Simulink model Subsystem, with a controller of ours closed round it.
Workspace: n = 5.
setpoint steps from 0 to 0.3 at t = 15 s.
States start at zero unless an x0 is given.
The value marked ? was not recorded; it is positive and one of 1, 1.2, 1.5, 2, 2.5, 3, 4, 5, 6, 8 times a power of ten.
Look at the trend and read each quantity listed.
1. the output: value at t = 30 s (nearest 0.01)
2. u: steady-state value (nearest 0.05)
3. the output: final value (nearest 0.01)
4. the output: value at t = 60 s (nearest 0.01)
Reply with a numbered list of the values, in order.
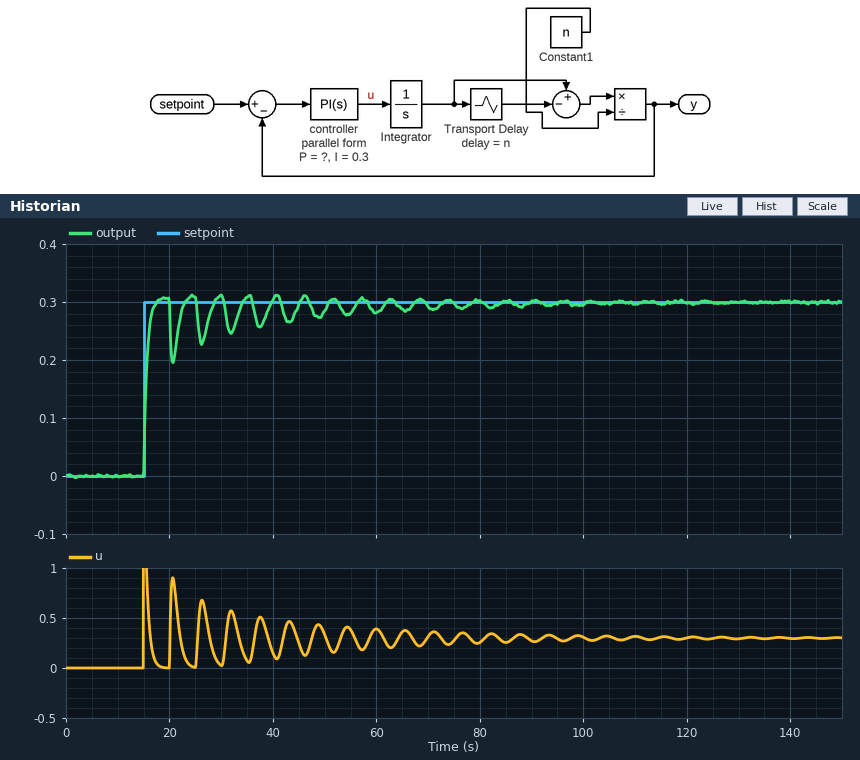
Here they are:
1. 0.31
2. 0.30
3. 0.30
4. 0.28
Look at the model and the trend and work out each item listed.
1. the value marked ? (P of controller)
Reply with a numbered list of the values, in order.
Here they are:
1. 8
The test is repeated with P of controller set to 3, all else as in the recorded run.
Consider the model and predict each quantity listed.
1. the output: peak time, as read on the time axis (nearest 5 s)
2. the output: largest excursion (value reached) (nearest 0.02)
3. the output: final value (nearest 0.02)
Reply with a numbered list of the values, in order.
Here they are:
1. 20 s
2. 0.32
3. 0.30
